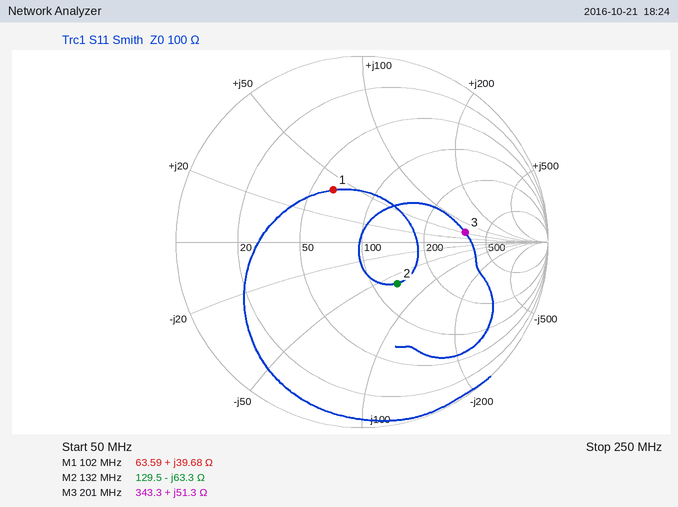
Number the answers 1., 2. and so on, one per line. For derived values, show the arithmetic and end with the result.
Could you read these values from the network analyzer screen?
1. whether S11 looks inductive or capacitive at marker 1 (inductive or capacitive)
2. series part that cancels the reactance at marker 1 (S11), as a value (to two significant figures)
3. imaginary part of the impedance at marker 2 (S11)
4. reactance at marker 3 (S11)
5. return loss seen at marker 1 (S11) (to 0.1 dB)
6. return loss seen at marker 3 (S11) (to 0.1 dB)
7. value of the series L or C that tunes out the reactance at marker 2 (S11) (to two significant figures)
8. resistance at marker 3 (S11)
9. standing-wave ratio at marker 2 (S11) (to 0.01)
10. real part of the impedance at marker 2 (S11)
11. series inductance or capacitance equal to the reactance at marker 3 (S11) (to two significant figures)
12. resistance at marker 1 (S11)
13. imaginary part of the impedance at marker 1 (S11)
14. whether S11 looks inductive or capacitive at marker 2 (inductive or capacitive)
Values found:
1. inductive
2. C = 1/(2π × 102 MHz × 39.68 Ω) ≈ 39 pF
3. -63.3 Ω
4. +51.3 Ω
5. 9.9 dB
6. 5.1 dB
7. L = 63.3 Ω/(2π × 132 MHz) ≈ 76 nH
8. 343.3 Ω
9. 1.83
10. 129.5 Ω
11. L = 51.3 Ω/(2π × 201 MHz) ≈ 41 nH
12. 63.59 Ω
13. +39.68 Ω
14. capacitive
